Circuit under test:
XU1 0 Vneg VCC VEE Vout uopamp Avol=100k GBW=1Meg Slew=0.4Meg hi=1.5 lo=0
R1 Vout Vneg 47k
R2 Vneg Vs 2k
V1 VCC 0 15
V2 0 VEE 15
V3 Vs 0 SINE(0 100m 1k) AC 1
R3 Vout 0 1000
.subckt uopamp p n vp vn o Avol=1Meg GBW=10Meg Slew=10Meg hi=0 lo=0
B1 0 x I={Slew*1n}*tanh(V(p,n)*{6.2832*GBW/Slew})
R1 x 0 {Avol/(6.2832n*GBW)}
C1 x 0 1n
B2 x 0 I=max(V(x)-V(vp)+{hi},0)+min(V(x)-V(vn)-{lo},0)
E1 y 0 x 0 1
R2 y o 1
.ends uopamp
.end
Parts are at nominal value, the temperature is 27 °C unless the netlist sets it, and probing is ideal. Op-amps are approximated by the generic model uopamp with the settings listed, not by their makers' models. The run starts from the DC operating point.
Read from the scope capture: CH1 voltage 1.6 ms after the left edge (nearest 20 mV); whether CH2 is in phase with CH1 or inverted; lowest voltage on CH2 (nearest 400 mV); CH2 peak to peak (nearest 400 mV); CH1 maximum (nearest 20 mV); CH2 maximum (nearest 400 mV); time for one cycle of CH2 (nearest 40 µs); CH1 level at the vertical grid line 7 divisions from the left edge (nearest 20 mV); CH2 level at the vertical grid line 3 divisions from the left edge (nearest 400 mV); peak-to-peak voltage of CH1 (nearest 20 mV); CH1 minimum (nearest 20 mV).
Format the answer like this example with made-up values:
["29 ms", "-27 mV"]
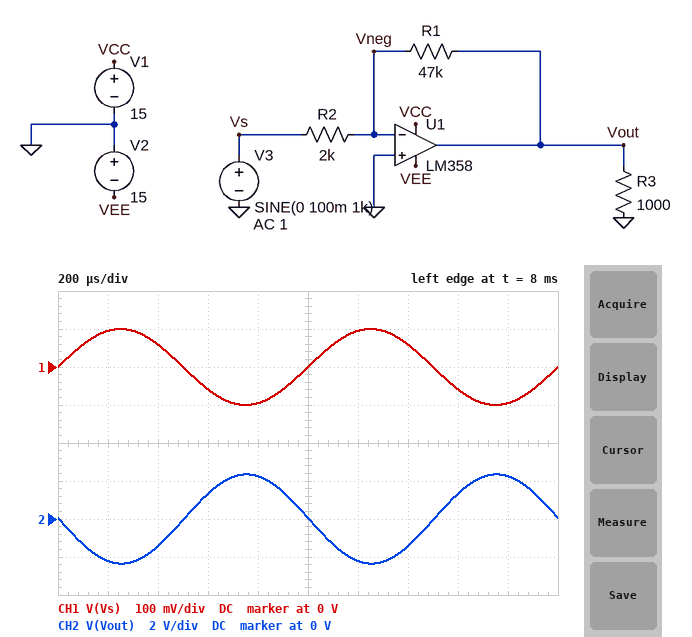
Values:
["-60 mV", "inverted", "-2.4 V", "4.8 V", "100 mV", "2.4 V", "1.00 ms", "60 mV", "1.2 V", "200 mV", "-100 mV"]
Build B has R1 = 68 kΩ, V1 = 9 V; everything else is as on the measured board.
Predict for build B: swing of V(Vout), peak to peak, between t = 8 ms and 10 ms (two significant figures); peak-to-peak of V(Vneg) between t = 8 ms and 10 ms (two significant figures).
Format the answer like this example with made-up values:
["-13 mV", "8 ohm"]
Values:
["6.8 V", "6.8 mV"]
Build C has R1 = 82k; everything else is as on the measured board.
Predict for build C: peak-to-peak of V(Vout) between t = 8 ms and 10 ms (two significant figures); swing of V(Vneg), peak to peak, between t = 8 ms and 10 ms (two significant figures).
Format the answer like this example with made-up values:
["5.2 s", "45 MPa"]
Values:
["8.2 V", "8.2 mV"]
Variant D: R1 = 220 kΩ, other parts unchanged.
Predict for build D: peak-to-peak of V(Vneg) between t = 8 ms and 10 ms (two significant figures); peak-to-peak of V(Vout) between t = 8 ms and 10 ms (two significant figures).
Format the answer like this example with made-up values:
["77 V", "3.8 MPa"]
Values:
["22 mV", "22 V"]
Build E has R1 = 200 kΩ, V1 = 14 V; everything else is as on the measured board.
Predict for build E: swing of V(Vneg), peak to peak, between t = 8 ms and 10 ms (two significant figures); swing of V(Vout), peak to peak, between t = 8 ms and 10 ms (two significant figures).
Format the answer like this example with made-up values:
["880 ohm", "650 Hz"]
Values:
["20 mV", "20 V"]
